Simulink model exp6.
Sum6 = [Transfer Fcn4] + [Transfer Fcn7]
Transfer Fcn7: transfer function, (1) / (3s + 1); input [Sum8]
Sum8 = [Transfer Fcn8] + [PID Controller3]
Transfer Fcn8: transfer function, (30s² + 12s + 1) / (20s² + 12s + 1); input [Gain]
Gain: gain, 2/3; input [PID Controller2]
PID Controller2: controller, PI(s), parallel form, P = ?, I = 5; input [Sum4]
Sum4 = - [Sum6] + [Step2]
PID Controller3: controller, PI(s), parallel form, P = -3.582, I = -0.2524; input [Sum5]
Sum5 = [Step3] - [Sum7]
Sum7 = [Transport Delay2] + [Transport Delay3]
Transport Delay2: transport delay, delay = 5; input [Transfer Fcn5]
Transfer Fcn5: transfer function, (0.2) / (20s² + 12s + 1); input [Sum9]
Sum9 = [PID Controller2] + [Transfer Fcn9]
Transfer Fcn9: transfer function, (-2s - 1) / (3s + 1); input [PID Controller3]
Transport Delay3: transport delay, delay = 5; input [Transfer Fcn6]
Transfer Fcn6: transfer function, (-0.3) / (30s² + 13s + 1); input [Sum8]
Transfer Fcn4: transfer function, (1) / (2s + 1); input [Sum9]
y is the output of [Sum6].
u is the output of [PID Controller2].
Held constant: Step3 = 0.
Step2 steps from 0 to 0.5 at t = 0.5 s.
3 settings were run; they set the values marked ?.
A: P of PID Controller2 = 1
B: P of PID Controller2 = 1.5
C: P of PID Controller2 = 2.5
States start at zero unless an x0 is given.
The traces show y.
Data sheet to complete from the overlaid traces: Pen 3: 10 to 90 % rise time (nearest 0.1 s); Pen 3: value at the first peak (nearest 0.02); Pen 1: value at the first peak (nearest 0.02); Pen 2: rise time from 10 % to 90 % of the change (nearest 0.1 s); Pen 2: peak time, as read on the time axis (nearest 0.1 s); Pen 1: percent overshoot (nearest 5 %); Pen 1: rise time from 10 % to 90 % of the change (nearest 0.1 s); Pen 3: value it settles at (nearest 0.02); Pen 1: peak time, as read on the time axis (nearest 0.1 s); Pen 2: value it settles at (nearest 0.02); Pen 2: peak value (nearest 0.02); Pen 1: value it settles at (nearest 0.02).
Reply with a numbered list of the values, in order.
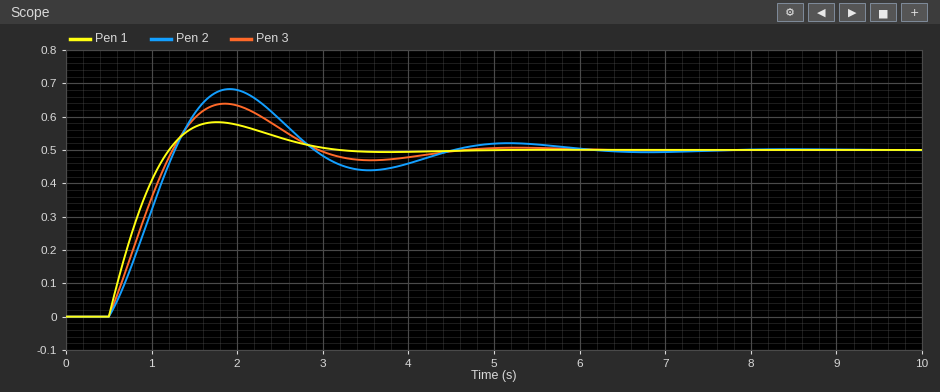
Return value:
1. 0.6 s
2. 0.64
3. 0.58
4. 0.6 s
5. 1.9 s
6. 15 %
7. 0.5 s
8. 0.50
9. 1.8 s
10. 0.50
11. 0.68
12. 0.50
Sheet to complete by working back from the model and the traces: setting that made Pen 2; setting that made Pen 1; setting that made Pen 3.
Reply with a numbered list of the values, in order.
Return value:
1. A
2. C
3. B
